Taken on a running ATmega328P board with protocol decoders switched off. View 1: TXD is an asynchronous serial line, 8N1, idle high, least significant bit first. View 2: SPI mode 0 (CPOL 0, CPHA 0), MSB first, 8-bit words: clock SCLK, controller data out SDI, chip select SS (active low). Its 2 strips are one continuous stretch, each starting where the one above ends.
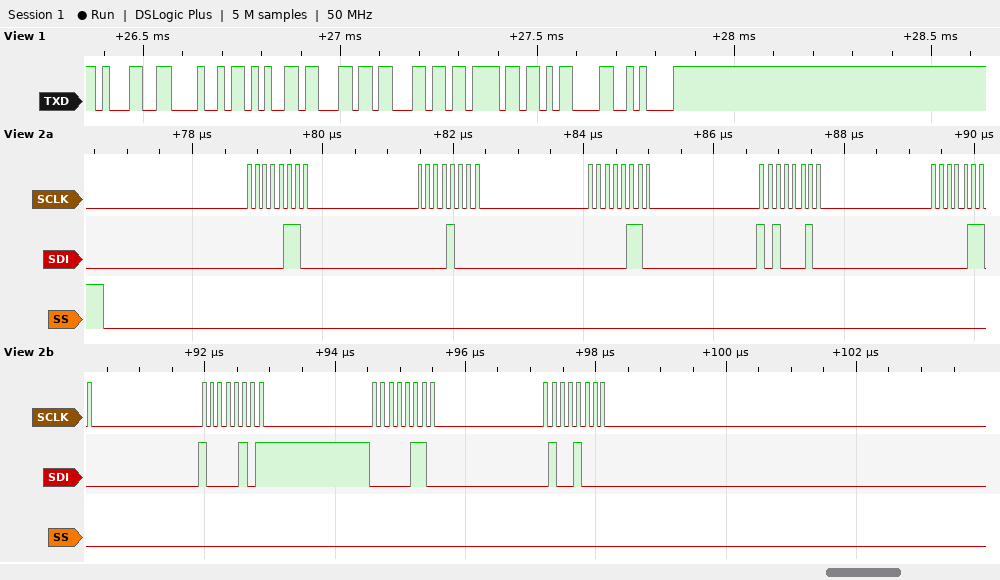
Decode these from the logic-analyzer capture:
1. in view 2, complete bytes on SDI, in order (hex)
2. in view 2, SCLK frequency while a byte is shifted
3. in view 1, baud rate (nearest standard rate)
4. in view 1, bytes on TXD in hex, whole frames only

06 08 06 A2 06 85 06 48
8 MHz
57600 baud
31 48 65 6C 6C 6F 0D 0A
